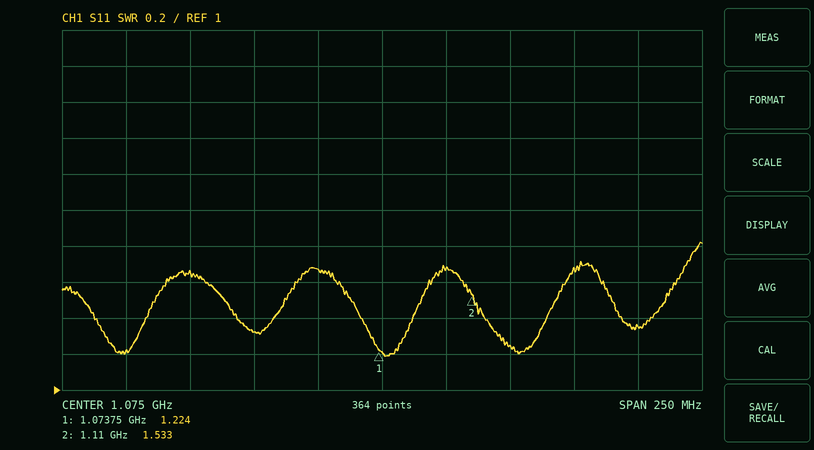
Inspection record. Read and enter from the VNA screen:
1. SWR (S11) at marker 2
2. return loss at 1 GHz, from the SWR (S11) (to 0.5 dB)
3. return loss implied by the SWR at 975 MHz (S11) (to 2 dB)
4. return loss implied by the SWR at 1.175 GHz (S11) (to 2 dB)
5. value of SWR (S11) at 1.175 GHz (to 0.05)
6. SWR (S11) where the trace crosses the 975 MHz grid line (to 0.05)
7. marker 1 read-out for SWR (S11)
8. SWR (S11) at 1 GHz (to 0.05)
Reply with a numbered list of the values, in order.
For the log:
1. 1.533
2. 12.0 dB
3. 20 dB
4. 16 dB
5. 1.35
6. 1.20
7. 1.224
8. 1.65
